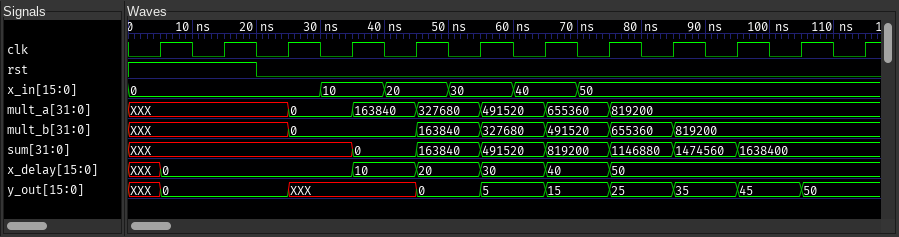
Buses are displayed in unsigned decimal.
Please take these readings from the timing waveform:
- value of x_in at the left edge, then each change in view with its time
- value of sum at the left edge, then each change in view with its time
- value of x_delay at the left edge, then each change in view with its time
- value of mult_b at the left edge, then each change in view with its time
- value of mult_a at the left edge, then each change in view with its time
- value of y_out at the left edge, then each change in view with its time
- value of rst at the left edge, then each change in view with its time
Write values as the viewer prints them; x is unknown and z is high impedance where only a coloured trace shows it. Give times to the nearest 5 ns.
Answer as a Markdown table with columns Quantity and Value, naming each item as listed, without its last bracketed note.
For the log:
| Quantity | Value |
|---|---|
| value of x_in at the left edge, then each change in view with its time | 0, 10 at 30 ns, 20 at 40 ns, 30 at 50 ns, 40 at 60 ns, 50 at 70 ns |
| value of sum at the left edge, then each change in view with its time | XXX, 0 at 35 ns, 163840 at 45 ns, 491520 at 55 ns, 819200 at 65 ns, 1146880 at 75 ns, 1474560 at 85 ns, 1638400 at 95 ns |
| value of x_delay at the left edge, then each change in view with its time | XXX, 0 at 5 ns, 10 at 35 ns, 20 at 45 ns, 30 at 55 ns, 40 at 65 ns, 50 at 75 ns |
| value of mult_b at the left edge, then each change in view with its time | XXX, 0 at 25 ns, 163840 at 45 ns, 327680 at 55 ns, 491520 at 65 ns, 655360 at 75 ns, 819200 at 85 ns |
| value of mult_a at the left edge, then each change in view with its time | XXX, 0 at 25 ns, 163840 at 35 ns, 327680 at 45 ns, 491520 at 55 ns, 655360 at 65 ns, 819200 at 75 ns |
| value of y_out at the left edge, then each change in view with its time | XXX, 0 at 5 ns, XXX at 25 ns, 0 at 45 ns, 5 at 55 ns, 15 at 65 ns, 25 at 75 ns, 35 at 85 ns, 45 at 95 ns, 50 at 105 ns |
| value of rst at the left edge, then each change in view with its time | 1, 0 at 20 ns |
